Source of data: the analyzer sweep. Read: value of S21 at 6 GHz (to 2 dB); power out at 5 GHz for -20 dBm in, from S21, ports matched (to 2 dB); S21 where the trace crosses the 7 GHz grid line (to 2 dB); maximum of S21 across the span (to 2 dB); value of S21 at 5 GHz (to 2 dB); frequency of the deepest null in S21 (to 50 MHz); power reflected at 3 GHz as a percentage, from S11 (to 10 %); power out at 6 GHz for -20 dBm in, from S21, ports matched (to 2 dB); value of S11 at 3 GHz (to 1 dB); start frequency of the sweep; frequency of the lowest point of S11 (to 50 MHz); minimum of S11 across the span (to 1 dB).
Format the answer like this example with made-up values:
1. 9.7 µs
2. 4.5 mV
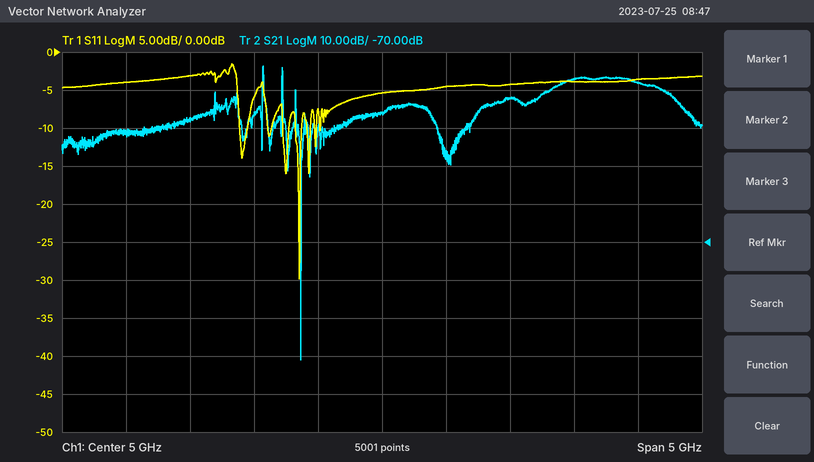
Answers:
1. -32 dB
2. -56 dBm
3. -28 dB
4. -24 dB
5. -36 dB
6. 4.35 GHz
7. 40 %
8. -52 dBm
9. -4 dB
10. 2.5 GHz
11. 4.35 GHz
12. -30 dB
